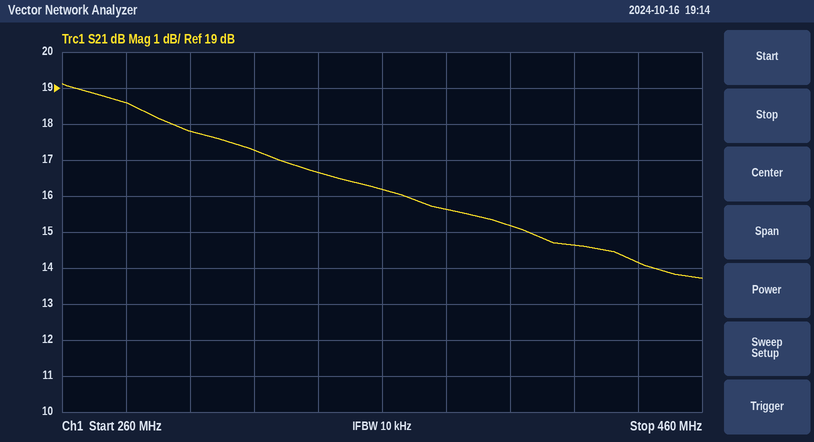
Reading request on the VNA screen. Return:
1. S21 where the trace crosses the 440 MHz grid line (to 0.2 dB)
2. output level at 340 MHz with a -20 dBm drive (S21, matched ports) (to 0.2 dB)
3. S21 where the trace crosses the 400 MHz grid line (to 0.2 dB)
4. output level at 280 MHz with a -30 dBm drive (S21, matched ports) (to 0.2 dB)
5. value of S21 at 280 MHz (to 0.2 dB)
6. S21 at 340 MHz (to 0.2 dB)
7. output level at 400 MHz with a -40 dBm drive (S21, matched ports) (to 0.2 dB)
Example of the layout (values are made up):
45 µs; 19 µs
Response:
14.2 dB; -3.4 dBm; 15.2 dB; -11.4 dBm; 18.6 dB; 16.6 dB; -24.8 dBm
